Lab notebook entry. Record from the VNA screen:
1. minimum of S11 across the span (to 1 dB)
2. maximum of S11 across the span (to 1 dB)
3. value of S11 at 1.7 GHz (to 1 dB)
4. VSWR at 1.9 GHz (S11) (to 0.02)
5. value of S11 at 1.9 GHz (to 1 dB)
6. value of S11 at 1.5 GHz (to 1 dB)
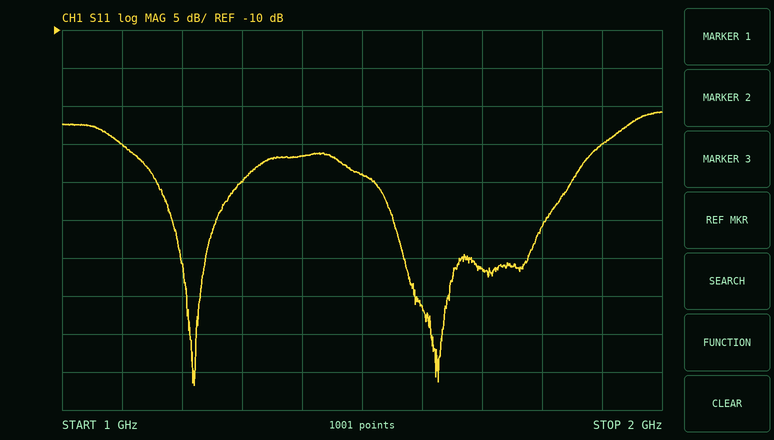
-57 dB
-21 dB
-41 dB
1.12
-25 dB
-29 dB
